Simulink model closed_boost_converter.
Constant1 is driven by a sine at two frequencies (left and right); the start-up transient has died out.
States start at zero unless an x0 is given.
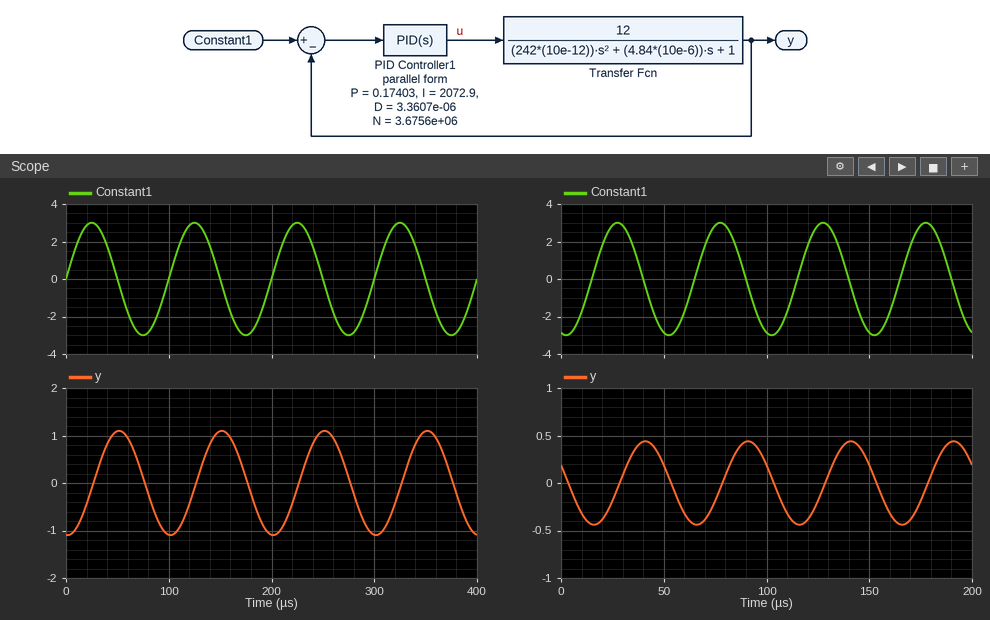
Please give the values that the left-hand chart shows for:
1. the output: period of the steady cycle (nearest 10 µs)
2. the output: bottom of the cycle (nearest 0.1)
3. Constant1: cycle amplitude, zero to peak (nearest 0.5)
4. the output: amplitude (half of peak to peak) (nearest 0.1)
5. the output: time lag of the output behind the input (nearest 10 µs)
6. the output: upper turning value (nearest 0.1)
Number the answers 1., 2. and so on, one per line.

1. 100 µs
2. -1.1
3. 3.0
4. 1.1
5. 30 µs
6. 1.1
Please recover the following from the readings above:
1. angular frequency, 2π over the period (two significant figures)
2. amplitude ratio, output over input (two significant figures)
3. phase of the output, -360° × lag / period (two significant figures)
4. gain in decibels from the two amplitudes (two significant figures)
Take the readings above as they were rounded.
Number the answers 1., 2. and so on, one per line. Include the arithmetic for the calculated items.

1. 2π / 100 = 0.063 rad/µs
2. 1.1 / 3 = 0.37
3. -360 × 30 / 100 = -110°
4. 20 log10(1.1 / 3) = -8.7 dB
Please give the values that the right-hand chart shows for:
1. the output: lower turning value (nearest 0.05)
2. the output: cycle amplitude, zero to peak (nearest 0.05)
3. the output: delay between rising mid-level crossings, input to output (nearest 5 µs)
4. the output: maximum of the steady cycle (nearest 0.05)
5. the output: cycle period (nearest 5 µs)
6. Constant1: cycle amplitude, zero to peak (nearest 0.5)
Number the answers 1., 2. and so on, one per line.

1. -0.45
2. 0.45
3. 15 µs
4. 0.45
5. 50 µs
6. 3.0
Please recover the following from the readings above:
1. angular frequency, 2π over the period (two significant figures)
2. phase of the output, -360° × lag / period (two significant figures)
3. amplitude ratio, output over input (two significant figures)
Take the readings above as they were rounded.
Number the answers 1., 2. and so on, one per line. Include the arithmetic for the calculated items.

1. 2π / 50 = 0.13 rad/µs
2. -360 × 15 / 50 = -110°
3. 0.45 / 3 = 0.15
